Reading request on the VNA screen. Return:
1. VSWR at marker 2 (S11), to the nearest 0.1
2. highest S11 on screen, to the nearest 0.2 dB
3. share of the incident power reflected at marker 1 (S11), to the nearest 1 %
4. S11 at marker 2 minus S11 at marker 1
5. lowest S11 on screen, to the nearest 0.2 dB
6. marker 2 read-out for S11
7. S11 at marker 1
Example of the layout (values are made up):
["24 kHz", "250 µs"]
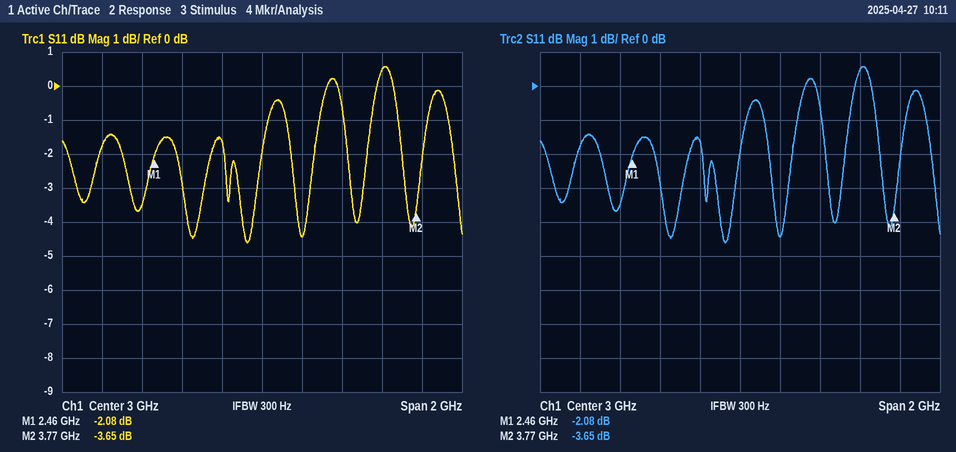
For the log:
["4.8", "0.6 dB", "62 %", "-1.57 dB", "-4.6 dB", "-3.65 dB", "-2.08 dB"]
